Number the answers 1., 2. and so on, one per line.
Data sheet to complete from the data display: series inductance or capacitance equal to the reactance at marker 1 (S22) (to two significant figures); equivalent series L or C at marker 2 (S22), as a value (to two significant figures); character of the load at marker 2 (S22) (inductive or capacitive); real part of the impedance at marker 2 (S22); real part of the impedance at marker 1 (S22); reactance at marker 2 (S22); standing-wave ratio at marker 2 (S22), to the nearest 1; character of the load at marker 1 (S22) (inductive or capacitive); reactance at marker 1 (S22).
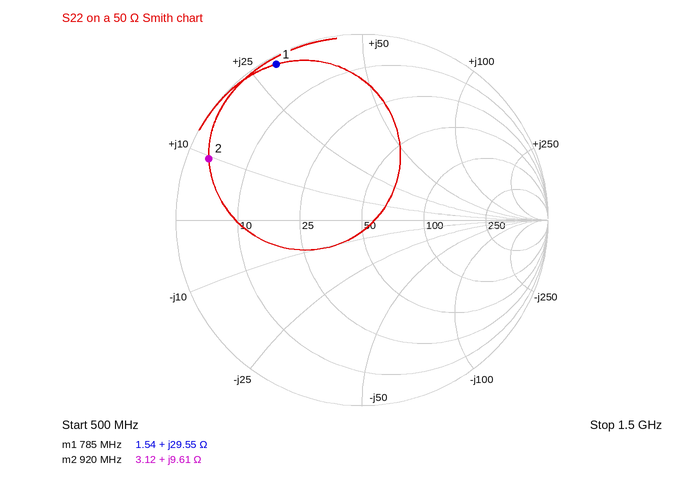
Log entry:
1. 6.0 nH
2. 1.7 nH
3. inductive
4. 3.12 Ω
5. 1.54 Ω
6. +9.61 Ω
7. 17
8. inductive
9. +29.55 Ω
